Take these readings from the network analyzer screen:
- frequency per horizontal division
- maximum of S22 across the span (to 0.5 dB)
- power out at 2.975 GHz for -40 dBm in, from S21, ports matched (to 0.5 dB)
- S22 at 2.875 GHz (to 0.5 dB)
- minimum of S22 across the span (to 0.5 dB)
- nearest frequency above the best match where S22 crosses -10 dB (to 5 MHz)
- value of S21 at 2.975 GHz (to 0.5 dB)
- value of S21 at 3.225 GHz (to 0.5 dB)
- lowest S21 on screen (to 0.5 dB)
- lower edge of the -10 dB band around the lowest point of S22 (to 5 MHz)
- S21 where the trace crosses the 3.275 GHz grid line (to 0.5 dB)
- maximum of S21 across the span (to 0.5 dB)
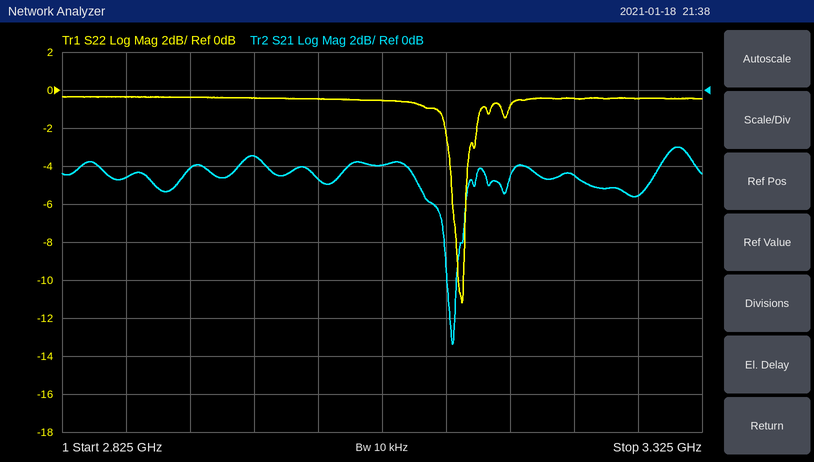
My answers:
50 MHz
-0.5 dB
-43.5 dBm
-0.5 dB
-11.0 dB
3.140 GHz
-3.5 dB
-4.5 dB
-13.5 dB
3.135 GHz
-5.5 dB
-3.0 dB
